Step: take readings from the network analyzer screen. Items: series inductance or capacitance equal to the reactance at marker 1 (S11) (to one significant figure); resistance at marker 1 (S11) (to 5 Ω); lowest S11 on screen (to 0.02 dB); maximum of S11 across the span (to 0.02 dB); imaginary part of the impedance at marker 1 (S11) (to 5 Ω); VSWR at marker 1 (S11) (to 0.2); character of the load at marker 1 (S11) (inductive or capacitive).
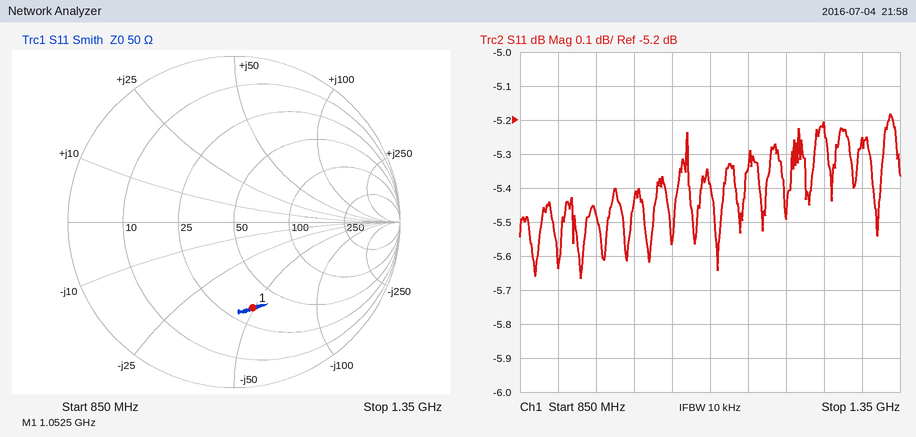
3 pF
35 Ω
-5.66 dB
-5.18 dB
-50 Ω
3.2
capacitive
